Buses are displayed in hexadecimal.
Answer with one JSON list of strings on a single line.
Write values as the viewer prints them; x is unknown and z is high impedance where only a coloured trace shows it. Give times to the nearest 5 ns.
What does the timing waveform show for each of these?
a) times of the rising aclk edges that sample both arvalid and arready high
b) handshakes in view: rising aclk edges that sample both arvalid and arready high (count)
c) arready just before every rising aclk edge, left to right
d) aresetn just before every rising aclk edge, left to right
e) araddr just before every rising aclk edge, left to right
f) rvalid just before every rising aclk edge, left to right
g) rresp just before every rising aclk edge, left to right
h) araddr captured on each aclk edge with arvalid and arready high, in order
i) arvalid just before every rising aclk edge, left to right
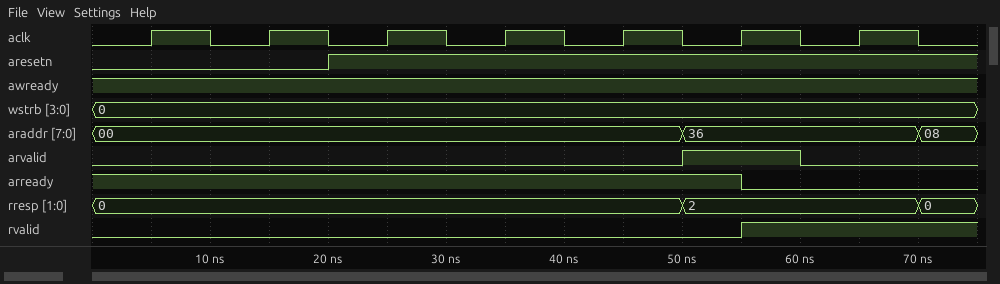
["55 ns", "1", "1 1 1 1 1 1 0", "0 0 1 1 1 1 1", "00, 00, 00, 00, 00, 36, 36", "0 0 0 0 0 0 1", "0, 0, 0, 0, 0, 2, 2", "36", "0 0 0 0 0 1 0"]
